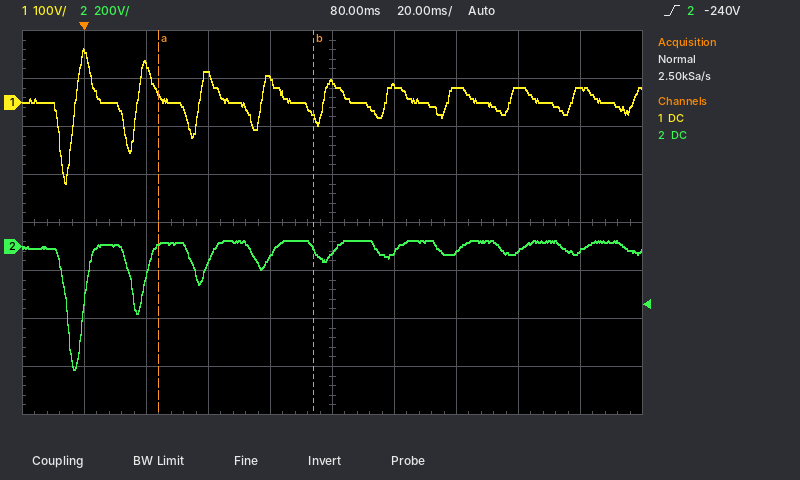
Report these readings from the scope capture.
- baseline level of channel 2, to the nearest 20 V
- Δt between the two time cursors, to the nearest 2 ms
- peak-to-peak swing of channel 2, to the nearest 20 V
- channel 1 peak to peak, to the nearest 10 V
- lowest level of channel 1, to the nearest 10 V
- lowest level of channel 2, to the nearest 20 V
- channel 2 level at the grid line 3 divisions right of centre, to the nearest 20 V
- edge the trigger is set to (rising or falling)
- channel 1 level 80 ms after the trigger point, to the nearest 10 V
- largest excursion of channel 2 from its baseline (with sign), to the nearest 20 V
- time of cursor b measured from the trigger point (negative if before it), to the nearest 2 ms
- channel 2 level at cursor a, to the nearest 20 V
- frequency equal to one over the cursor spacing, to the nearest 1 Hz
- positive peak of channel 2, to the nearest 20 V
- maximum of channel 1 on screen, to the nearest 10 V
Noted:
0 V
50 ms
540 V
280 V
-170 V
-520 V
-20 V
rising
40 V
-520 V
+74 ms
0 V
20 Hz
20 V
110 V
